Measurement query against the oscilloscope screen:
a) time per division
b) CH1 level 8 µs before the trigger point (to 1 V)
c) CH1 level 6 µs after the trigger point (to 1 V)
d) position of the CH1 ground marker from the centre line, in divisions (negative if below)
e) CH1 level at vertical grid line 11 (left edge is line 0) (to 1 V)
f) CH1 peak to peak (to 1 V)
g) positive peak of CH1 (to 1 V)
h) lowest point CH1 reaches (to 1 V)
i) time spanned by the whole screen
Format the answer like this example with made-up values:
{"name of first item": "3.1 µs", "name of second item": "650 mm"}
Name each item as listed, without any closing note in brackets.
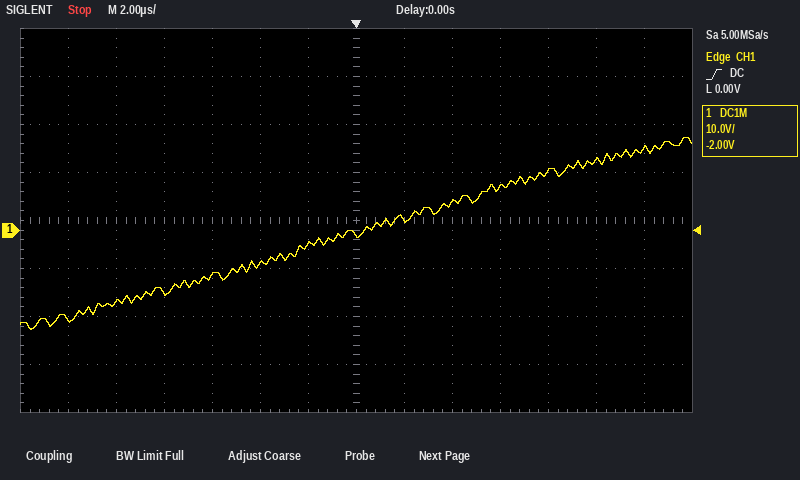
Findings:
{"time per division": "2 µs", "CH1 level 8 µs before the trigger point": "-13 V", "CH1 level 6 µs after the trigger point": "9 V", "position of the CH1 ground marker from the centre line, in divisions": "-0.2 div", "CH1 level at vertical grid line 11 (left edge is line 0)": "12 V", "CH1 peak to peak": "40 V", "positive peak of CH1": "19 V", "lowest point CH1 reaches": "-21 V", "time spanned by the whole screen": "28 µs"}
